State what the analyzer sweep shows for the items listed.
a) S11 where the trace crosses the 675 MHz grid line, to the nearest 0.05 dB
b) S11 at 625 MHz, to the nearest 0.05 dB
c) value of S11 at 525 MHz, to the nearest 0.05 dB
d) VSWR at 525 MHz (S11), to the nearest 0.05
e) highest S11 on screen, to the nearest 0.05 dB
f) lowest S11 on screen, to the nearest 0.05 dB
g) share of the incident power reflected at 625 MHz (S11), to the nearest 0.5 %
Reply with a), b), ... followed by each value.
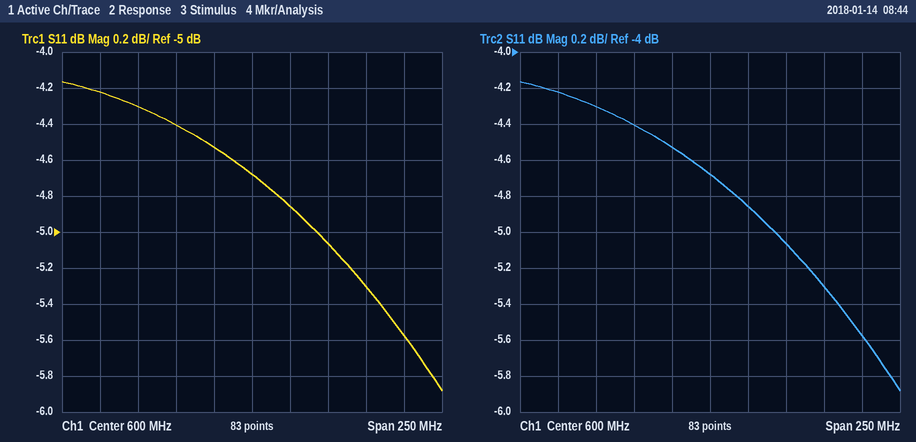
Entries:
a) -5.30 dB
b) -4.85 dB
c) -4.30 dB
d) 4.10
e) -4.15 dB
f) -5.90 dB
g) 32.5 %
